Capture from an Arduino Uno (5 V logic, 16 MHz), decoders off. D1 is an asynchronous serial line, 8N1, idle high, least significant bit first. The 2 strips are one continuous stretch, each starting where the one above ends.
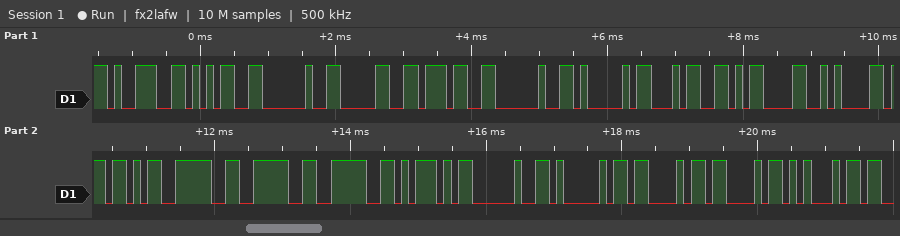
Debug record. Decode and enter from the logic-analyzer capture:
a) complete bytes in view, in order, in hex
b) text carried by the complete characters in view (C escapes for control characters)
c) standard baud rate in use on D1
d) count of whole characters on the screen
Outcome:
39 35 20 30 37 20 41 34 0D 0A 5B 3E 3E 3E 5D 20 41 43 43 45
"95 07 A4\r\n[>>>] ACCE"
9600 baud
20
